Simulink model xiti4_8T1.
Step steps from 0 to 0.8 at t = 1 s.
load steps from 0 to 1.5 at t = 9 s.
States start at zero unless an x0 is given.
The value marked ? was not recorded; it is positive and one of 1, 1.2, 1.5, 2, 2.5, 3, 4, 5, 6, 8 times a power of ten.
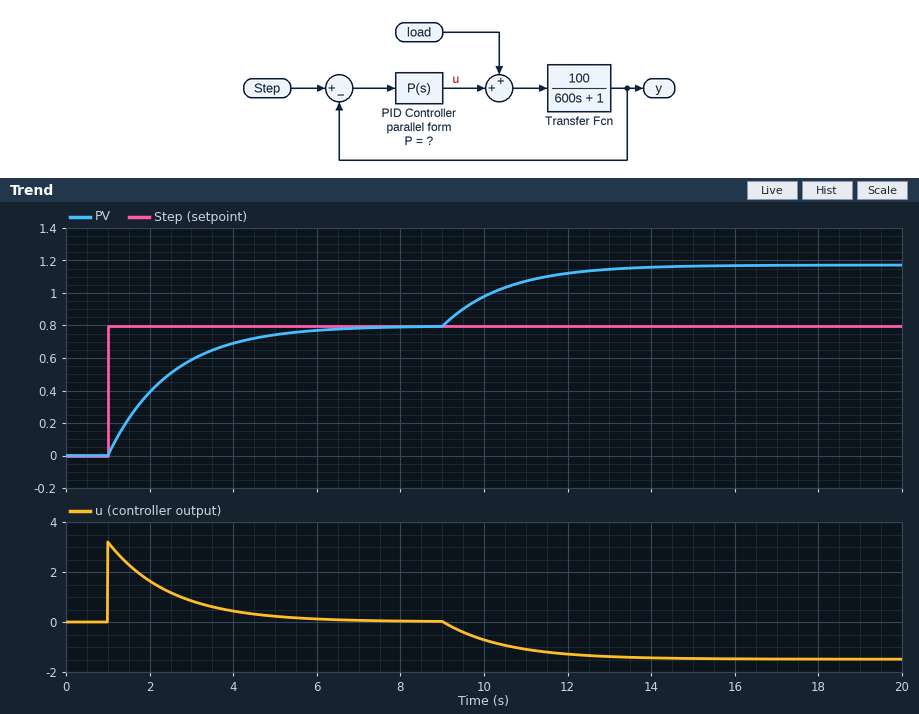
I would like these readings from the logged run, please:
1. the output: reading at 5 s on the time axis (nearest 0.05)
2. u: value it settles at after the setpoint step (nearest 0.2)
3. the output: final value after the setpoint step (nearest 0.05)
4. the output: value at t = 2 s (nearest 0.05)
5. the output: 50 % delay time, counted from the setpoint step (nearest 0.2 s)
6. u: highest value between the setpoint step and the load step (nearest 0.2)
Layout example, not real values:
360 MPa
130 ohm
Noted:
0.75
0.0
0.80
0.40
1.0 s
3.2
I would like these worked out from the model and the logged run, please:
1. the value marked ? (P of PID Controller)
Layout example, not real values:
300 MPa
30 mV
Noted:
4
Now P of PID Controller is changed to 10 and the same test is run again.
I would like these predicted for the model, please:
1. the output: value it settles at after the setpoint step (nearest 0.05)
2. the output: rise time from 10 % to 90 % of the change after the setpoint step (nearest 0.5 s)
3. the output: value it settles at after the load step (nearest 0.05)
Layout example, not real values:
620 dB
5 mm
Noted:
0.80
1.5 s
0.95
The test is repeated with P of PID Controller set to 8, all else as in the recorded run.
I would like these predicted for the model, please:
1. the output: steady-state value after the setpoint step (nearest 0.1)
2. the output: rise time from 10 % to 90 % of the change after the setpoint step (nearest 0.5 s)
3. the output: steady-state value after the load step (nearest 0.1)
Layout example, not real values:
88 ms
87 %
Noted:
0.8
1.5 s
1.0
